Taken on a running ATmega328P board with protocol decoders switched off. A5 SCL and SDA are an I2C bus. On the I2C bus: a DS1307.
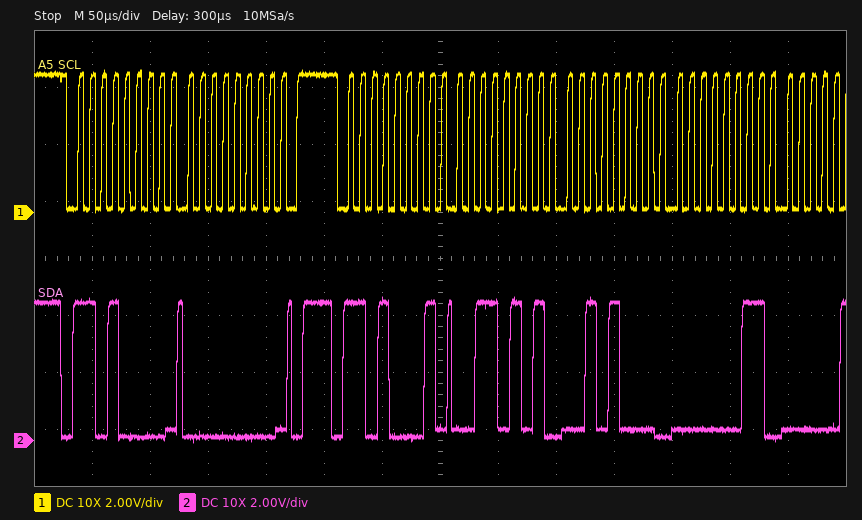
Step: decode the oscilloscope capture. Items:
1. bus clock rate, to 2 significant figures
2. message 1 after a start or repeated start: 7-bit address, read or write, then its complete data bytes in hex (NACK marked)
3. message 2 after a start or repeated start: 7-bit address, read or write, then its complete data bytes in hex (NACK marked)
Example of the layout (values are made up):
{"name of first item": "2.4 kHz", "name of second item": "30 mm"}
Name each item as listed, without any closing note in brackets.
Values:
{"bus clock rate, to 2 significant figures": "100 kHz", "message 1 after a start or repeated start: 7-bit address, read or write, then its complete data bytes in hex": "0x68 write: 00", "message 2 after a start or repeated start: 7-bit address, read or write, then its complete data bytes in hex": "0x68 read: 35 28 03"}
